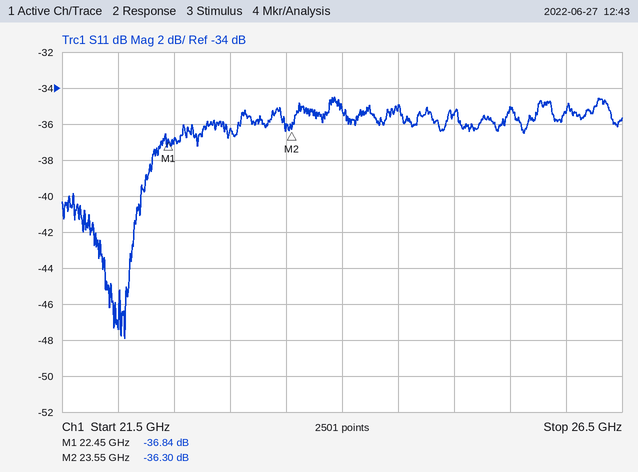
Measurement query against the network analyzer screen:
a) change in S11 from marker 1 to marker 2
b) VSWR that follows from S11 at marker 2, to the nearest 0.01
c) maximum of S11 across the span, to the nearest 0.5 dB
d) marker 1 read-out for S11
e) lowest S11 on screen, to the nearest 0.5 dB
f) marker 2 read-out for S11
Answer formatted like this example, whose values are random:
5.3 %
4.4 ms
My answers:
0.54 dB
1.03
-34.5 dB
-36.84 dB
-48.0 dB
-36.30 dB
